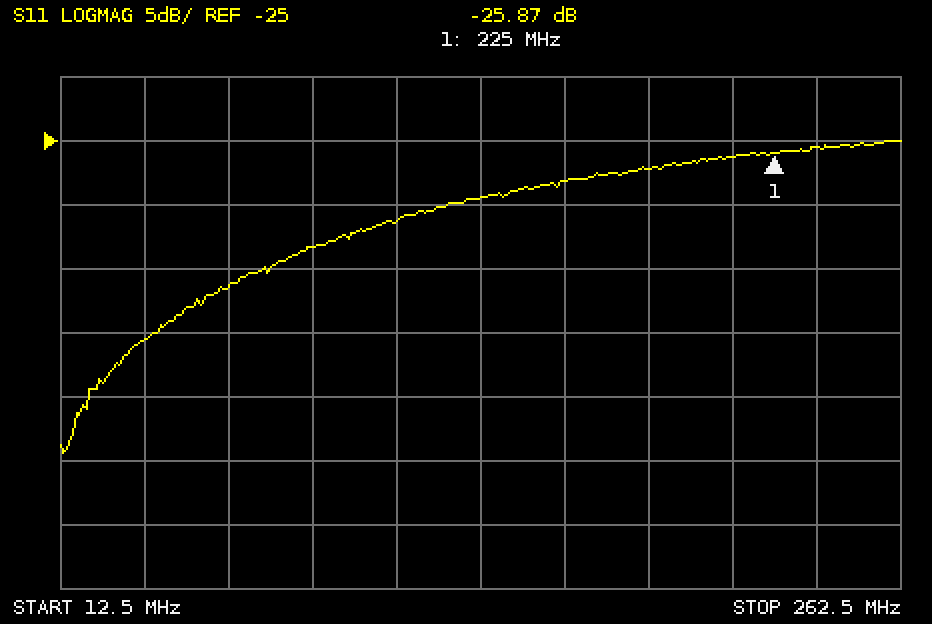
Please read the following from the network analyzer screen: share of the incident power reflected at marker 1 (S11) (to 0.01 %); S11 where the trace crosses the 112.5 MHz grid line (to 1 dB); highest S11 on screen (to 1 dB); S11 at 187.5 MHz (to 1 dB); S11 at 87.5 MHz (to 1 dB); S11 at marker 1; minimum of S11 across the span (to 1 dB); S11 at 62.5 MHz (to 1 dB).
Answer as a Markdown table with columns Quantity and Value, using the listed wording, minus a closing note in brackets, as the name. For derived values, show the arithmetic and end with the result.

| Quantity | Value |
|---|---|
| share of the incident power reflected at marker 1 (S11) | 10^(-25.87/10) ≈ 0.26 % |
| S11 where the trace crosses the 112.5 MHz grid line | -31 dB |
| highest S11 on screen | -25 dB |
| S11 at 187.5 MHz | -27 dB |
| S11 at 87.5 MHz | -33 dB |
| S11 at marker 1 | -25.87 dB |
| minimum of S11 across the span | -49 dB |
| S11 at 62.5 MHz | -36 dB |
